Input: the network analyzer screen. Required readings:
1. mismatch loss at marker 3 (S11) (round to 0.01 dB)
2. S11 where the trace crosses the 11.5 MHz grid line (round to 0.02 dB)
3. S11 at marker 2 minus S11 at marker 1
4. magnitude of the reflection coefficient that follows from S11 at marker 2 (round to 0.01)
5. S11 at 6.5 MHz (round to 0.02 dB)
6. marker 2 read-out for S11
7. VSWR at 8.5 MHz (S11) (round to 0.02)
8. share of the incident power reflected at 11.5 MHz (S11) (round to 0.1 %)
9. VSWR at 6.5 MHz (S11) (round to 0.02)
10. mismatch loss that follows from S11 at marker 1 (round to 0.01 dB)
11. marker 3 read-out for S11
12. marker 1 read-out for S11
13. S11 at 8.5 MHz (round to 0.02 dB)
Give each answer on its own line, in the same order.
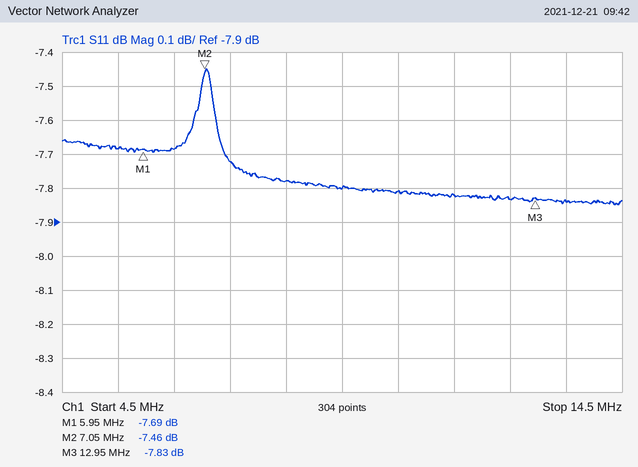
0.78 dB
-7.82 dB
0.23 dB
0.42
-7.68 dB
-7.46 dB
2.38
16.5 %
2.40
0.81 dB
-7.83 dB
-7.69 dB
-7.78 dB
